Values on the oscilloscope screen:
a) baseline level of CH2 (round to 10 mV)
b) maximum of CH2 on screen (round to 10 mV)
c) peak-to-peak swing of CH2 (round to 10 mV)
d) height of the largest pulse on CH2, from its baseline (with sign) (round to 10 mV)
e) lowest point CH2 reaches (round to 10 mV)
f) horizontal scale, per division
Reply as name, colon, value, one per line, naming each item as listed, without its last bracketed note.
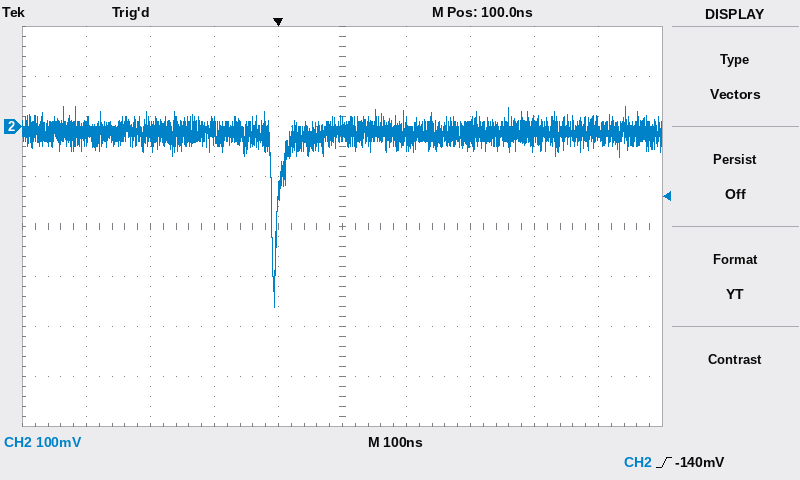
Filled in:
baseline level of CH2: -10 mV
maximum of CH2 on screen: 40 mV
peak-to-peak swing of CH2: 400 mV
height of the largest pulse on CH2, from its baseline (with sign): -350 mV
lowest point CH2 reaches: -360 mV
horizontal scale, per division: 100 ns
